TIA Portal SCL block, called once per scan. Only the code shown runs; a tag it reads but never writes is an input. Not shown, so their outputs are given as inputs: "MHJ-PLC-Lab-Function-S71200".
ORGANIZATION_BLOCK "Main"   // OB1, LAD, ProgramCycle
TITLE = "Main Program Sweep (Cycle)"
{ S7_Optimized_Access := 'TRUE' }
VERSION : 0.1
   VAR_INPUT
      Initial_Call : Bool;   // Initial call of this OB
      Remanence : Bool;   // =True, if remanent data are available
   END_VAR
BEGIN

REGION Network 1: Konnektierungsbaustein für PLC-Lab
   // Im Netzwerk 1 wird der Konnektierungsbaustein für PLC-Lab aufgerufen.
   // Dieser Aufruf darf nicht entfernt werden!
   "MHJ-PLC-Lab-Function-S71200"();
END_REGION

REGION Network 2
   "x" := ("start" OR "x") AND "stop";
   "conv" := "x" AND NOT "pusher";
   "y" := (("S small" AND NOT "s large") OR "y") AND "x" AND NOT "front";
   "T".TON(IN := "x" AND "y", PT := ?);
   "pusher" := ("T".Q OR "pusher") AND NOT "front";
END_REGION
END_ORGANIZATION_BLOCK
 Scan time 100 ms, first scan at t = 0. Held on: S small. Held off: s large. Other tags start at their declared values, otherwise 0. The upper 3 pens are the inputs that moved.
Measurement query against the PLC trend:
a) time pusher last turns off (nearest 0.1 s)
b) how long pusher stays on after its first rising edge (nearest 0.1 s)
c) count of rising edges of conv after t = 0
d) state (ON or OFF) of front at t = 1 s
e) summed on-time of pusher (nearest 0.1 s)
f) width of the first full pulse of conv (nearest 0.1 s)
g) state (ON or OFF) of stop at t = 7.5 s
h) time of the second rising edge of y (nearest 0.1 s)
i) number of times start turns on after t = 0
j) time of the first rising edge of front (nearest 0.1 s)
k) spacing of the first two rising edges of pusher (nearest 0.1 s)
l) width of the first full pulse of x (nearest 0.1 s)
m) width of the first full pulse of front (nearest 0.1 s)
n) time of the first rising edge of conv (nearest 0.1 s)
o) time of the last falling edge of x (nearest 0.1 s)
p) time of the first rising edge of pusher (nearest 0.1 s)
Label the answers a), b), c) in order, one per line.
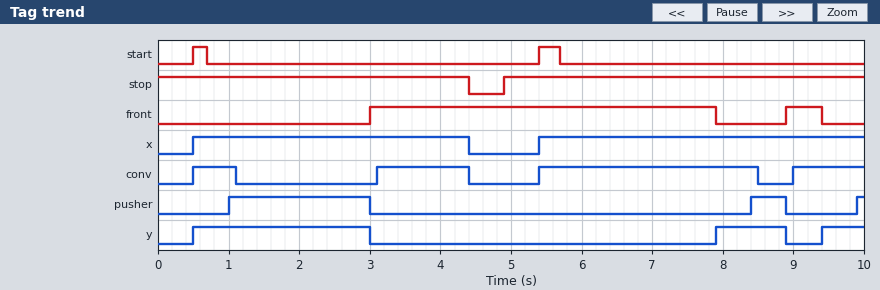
a) 8.9 s
b) 2.0 s
c) 4
d) OFF
e) 2.6 s
f) 0.6 s
g) ON
h) 7.9 s
i) 2
j) 3.0 s
k) 7.4 s
l) 3.9 s
m) 4.9 s
n) 0.5 s
o) 4.4 s
p) 1.0 s
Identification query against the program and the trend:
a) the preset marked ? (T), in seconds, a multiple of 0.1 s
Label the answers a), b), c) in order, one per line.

a) 0.5 s
